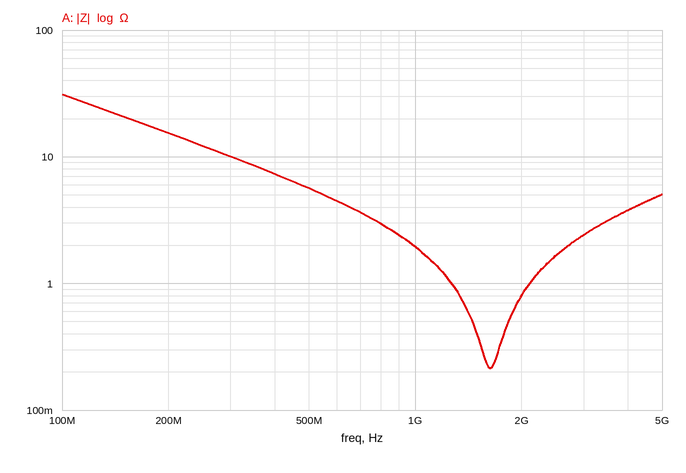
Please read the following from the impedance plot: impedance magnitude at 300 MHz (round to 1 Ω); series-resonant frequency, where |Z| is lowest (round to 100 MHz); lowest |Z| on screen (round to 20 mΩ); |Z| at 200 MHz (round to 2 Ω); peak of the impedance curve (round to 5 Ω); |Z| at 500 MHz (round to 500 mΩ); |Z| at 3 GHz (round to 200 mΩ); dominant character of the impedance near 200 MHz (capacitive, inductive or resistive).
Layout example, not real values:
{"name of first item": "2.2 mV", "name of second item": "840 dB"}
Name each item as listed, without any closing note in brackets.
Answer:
{"impedance magnitude at 300 MHz": "10 Ω", "series-resonant frequency, where |Z| is lowest": "1.6 GHz", "lowest |Z| on screen": "220 mΩ", "|Z| at 200 MHz": "16 Ω", "peak of the impedance curve": "30 Ω", "|Z| at 500 MHz": "5.5 Ω", "|Z| at 3 GHz": "2.4 Ω", "dominant character of the impedance near 200 MHz": "capacitive"}
